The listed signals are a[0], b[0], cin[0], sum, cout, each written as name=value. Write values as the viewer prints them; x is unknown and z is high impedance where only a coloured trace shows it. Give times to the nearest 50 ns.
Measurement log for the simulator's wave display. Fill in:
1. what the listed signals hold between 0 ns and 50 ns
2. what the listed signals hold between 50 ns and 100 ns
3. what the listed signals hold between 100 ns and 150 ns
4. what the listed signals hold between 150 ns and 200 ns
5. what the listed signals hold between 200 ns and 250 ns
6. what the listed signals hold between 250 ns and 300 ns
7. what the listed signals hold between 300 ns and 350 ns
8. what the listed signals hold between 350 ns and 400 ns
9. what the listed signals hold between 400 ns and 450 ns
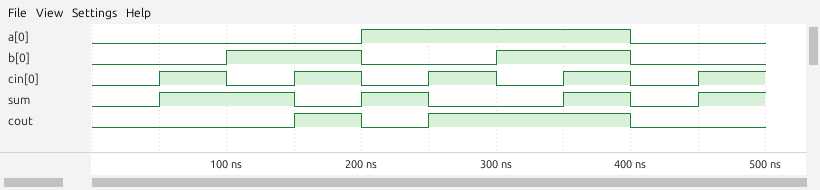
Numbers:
a[0]=0, b[0]=0, cin[0]=0, sum=0, cout=0
a[0]=0, b[0]=0, cin[0]=1, sum=1, cout=0
a[0]=0, b[0]=1, cin[0]=0, sum=1, cout=0
a[0]=0, b[0]=1, cin[0]=1, sum=0, cout=1
a[0]=1, b[0]=0, cin[0]=0, sum=1, cout=0
a[0]=1, b[0]=0, cin[0]=1, sum=0, cout=1
a[0]=1, b[0]=1, cin[0]=0, sum=0, cout=1
a[0]=1, b[0]=1, cin[0]=1, sum=1, cout=1
a[0]=0, b[0]=0, cin[0]=0, sum=0, cout=0
